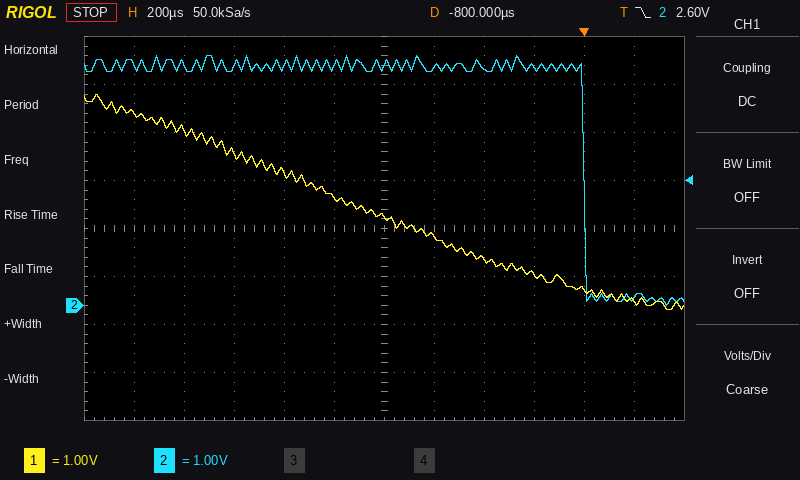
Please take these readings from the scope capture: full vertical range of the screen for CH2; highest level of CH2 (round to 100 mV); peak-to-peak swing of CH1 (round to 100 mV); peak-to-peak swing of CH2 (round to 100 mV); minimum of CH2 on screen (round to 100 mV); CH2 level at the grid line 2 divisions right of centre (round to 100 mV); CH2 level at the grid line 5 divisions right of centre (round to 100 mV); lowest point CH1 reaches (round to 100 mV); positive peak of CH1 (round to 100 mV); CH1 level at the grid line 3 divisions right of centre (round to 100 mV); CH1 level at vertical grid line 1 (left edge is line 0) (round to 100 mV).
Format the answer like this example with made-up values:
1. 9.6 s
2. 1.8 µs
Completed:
1. 8 V
2. 5.2 V
3. 4.5 V
4. 5.2 V
5. 0.0 V
6. 4.9 V
7. 200 mV
8. -100 mV
9. 4.4 V
10. 600 mV
11. 4.0 V
